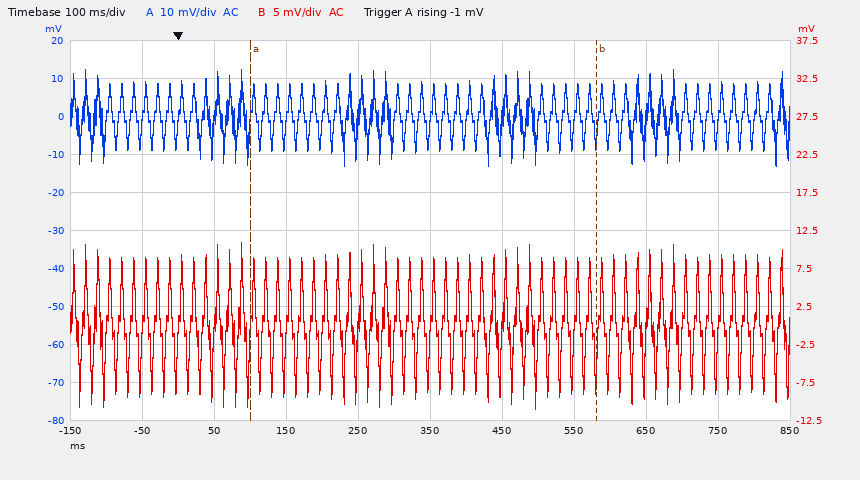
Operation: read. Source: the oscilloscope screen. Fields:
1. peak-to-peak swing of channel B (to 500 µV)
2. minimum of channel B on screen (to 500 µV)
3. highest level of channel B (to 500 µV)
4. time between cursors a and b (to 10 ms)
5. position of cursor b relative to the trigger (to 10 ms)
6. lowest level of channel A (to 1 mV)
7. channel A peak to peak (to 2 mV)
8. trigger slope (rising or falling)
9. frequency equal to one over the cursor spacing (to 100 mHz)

22.0 mV
-11.0 mV
11.0 mV
480 ms
+580 ms
-13 mV
26 mV
rising
2.1 Hz
